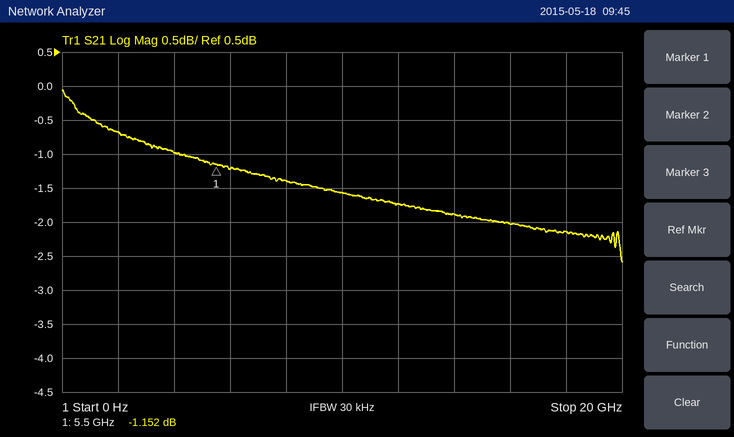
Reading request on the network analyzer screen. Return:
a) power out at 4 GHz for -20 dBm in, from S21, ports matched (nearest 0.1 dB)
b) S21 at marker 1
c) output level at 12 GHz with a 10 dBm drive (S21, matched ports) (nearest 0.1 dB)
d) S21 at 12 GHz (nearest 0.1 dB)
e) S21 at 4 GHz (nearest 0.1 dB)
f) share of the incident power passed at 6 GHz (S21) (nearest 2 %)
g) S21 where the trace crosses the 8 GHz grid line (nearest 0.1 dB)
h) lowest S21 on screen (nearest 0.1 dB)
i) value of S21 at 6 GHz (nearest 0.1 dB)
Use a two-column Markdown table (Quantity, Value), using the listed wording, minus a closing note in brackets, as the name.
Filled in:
| Quantity | Value |
|---|---|
| power out at 4 GHz for -20 dBm in, from S21, ports matched | -21.0 dBm |
| S21 at marker 1 | -1.152 dB |
| output level at 12 GHz with a 10 dBm drive (S21, matched ports) | 8.3 dBm |
| S21 at 12 GHz | -1.7 dB |
| S21 at 4 GHz | -1.0 dB |
| share of the incident power passed at 6 GHz (S21) | 76 % |
| S21 where the trace crosses the 8 GHz grid line | -1.4 dB |
| lowest S21 on screen | -2.6 dB |
| value of S21 at 6 GHz | -1.2 dB |
